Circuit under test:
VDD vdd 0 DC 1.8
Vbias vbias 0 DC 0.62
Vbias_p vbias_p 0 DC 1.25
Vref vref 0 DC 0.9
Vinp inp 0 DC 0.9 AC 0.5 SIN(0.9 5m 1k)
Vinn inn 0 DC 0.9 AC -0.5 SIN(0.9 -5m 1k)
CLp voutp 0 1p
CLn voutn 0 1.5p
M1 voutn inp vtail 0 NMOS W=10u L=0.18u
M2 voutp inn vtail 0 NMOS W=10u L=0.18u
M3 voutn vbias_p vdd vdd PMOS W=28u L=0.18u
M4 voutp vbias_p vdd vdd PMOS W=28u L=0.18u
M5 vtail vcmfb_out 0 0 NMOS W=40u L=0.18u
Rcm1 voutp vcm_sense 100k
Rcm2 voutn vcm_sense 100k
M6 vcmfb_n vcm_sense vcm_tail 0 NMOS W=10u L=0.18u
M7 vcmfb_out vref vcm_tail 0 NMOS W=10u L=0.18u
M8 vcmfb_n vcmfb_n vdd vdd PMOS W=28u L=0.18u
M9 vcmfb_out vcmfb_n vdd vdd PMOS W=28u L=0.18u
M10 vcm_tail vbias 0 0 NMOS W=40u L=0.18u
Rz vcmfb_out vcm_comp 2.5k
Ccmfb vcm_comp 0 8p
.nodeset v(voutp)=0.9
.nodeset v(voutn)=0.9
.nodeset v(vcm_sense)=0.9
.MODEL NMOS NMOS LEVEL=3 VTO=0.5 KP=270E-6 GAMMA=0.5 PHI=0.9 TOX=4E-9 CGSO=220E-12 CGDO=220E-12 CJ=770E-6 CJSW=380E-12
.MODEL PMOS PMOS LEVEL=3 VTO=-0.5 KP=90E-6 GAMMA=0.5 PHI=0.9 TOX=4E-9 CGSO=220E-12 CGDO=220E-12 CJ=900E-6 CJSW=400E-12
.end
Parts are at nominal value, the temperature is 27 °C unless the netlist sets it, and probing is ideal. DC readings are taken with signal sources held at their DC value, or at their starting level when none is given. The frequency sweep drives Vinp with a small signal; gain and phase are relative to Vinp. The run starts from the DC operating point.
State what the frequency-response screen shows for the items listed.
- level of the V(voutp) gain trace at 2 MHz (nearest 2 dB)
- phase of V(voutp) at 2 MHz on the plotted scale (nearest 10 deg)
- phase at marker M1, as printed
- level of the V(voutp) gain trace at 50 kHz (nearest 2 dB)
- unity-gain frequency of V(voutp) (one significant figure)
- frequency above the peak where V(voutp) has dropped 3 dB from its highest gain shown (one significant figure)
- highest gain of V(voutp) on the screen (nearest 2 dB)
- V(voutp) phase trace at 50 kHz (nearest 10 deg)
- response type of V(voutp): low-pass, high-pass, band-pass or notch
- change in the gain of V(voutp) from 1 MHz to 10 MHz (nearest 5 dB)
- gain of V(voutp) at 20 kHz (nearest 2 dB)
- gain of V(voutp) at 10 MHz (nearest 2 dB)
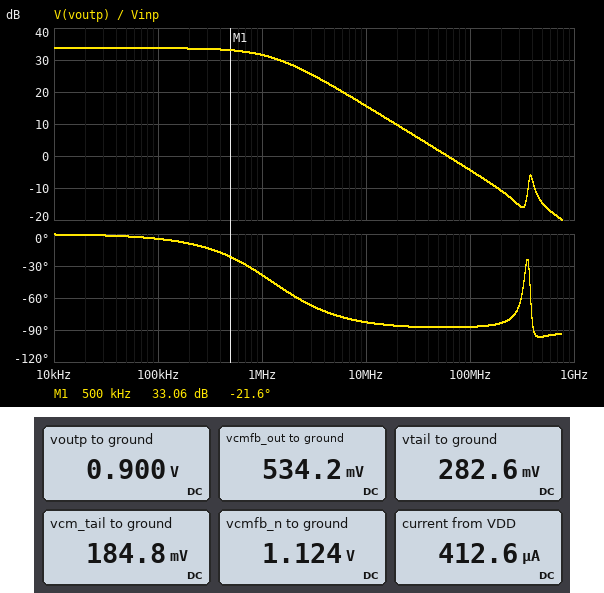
28 dB
-60 deg
-21.6 deg
34 dB
60 MHz
1 MHz
34 dB
0 deg
low-pass
-15 dB
34 dB
16 dB
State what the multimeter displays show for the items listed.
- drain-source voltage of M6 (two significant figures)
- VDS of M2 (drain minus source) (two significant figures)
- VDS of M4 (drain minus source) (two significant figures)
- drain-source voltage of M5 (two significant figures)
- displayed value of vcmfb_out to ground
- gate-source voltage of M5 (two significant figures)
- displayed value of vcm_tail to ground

940 mV
620 mV
-900 mV
280 mV
534.2 mV
530 mV
184.8 mV
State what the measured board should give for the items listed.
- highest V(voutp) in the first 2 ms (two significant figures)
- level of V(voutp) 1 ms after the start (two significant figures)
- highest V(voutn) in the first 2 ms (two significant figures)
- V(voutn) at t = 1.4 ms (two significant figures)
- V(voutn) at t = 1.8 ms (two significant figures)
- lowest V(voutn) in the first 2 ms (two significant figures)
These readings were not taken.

1.2 V
900 mV
1.2 V
710 mV
1.2 V
580 mV
